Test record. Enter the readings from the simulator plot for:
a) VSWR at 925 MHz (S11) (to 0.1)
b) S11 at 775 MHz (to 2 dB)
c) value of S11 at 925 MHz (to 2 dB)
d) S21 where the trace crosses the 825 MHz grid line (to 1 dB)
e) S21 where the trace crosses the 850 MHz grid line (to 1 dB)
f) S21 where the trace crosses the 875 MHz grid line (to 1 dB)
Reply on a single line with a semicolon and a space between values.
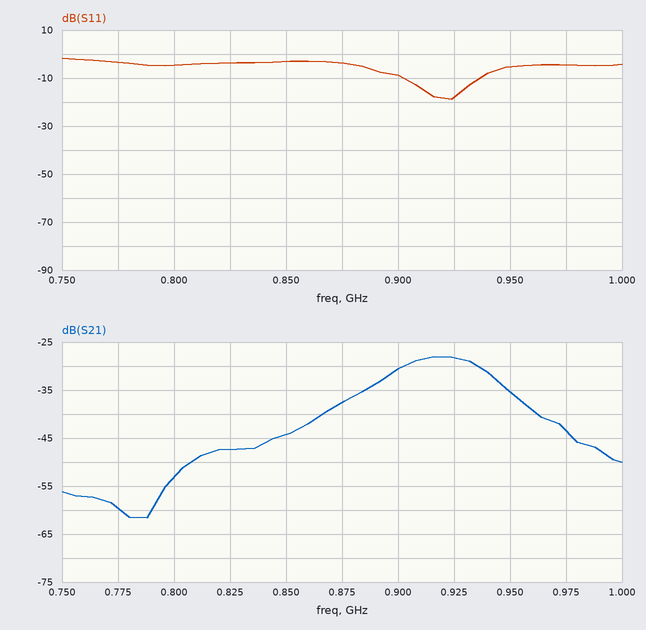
1.3; -4 dB; -18 dB; -47 dB; -44 dB; -38 dB
